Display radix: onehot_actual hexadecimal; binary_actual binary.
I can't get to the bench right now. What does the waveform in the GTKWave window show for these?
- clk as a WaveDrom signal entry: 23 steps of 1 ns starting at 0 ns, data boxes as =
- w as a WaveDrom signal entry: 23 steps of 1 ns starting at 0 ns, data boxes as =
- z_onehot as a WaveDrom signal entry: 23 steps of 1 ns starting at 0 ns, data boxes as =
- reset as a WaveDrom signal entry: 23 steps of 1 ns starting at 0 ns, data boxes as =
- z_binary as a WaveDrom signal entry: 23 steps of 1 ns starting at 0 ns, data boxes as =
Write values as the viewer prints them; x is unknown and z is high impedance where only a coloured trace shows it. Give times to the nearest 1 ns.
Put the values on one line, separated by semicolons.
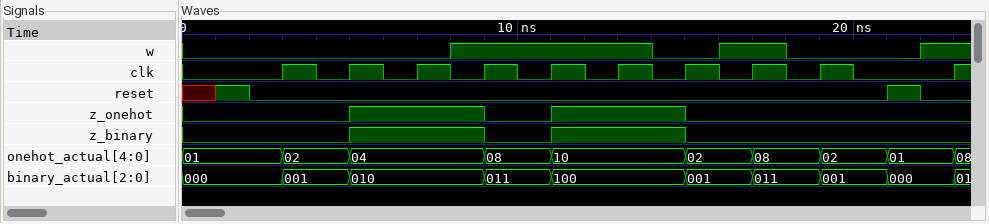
{name: 'clk', wave: '0..101010101010101010..'}; {name: 'w', wave: '0.......1.....0.1.0...1'}; {name: 'z_onehot', wave: '0....1...0.1...0.......'}; {name: 'reset', wave: 'x10..................10'}; {name: 'z_binary', wave: '0....1...0.1...0.......'}
